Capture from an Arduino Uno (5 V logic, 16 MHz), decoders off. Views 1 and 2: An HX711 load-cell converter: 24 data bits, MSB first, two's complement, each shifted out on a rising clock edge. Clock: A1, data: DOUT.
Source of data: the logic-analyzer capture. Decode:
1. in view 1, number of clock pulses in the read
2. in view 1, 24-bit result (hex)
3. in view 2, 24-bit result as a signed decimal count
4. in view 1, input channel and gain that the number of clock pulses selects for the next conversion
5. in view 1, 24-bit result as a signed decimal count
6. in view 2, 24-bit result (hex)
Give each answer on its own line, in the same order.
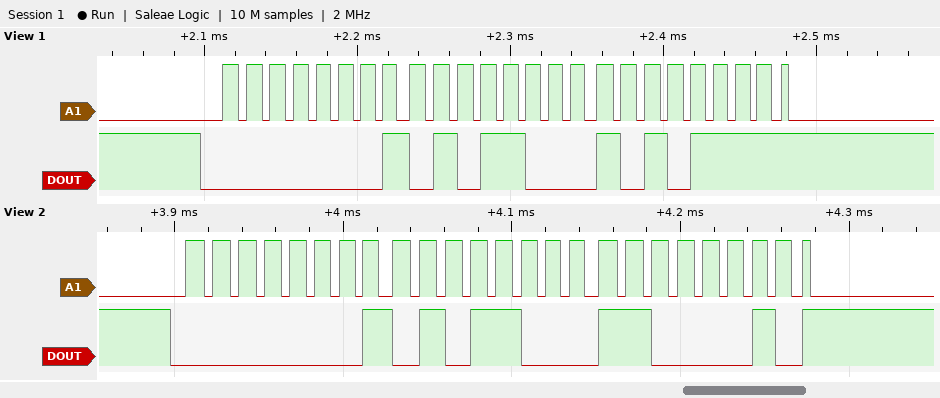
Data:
25
0x0158AF
88258
channel A, gain 128
88239
0x0158C2
